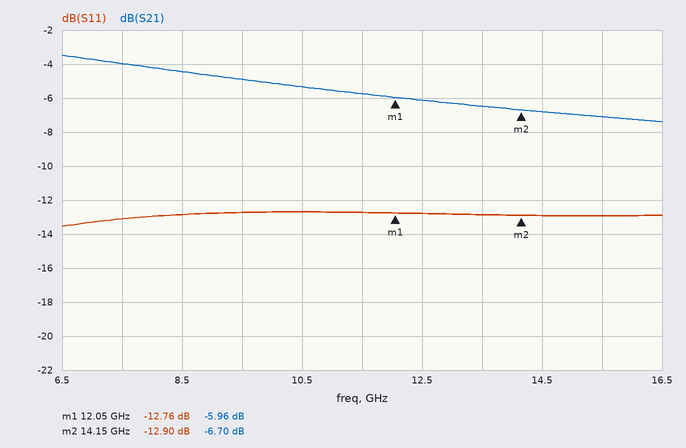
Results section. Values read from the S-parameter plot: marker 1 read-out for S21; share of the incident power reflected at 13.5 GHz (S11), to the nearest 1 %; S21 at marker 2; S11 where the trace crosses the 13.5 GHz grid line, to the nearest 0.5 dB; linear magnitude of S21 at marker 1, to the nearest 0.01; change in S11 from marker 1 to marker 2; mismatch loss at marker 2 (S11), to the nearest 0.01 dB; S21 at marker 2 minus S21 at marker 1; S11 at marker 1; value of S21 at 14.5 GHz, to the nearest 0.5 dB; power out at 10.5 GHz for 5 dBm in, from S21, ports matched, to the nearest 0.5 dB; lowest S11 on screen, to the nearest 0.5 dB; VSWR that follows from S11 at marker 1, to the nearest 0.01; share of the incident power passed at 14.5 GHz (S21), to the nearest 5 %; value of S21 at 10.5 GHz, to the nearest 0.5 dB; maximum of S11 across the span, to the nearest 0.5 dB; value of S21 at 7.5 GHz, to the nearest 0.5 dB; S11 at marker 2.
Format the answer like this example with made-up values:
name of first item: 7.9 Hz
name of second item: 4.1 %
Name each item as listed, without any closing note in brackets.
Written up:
marker 1 read-out for S21: -5.96 dB
share of the incident power reflected at 13.5 GHz (S11), to the nearest 1 %: 5 %
S21 at marker 2: -6.70 dB
S11 where the trace crosses the 13.5 GHz grid line, to the nearest 0.5 dB: -13.0 dB
linear magnitude of S21 at marker 1, to the nearest 0.01: 0.50
change in S11 from marker 1 to marker 2: -0.14 dB
mismatch loss at marker 2 (S11), to the nearest 0.01 dB: 0.23 dB
S21 at marker 2 minus S21 at marker 1: -0.74 dB
S11 at marker 1: -12.76 dB
value of S21 at 14.5 GHz, to the nearest 0.5 dB: -7.0 dB
power out at 10.5 GHz for 5 dBm in, from S21, ports matched, to the nearest 0.5 dB: -0.5 dBm
lowest S11 on screen, to the nearest 0.5 dB: -13.5 dB
VSWR that follows from S11 at marker 1, to the nearest 0.01: 1.60
share of the incident power passed at 14.5 GHz (S21), to the nearest 5 %: 20 %
value of S21 at 10.5 GHz, to the nearest 0.5 dB: -5.5 dB
maximum of S11 across the span, to the nearest 0.5 dB: -12.5 dB
value of S21 at 7.5 GHz, to the nearest 0.5 dB: -4.0 dB
S11 at marker 2: -12.90 dB
